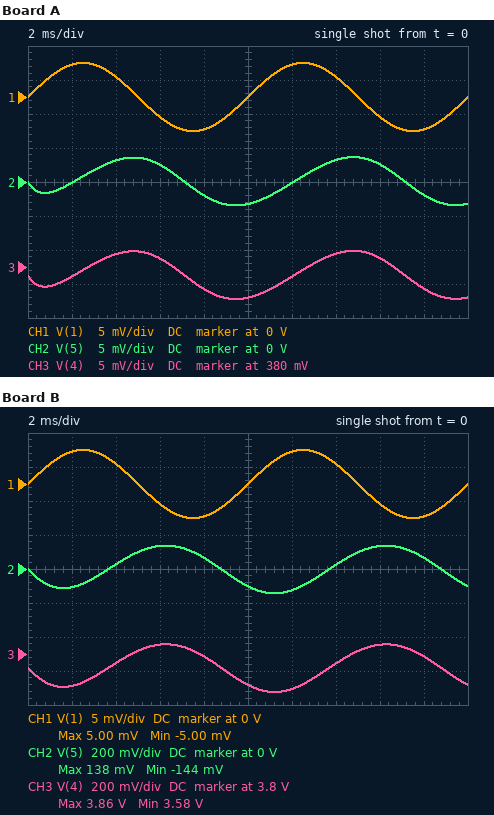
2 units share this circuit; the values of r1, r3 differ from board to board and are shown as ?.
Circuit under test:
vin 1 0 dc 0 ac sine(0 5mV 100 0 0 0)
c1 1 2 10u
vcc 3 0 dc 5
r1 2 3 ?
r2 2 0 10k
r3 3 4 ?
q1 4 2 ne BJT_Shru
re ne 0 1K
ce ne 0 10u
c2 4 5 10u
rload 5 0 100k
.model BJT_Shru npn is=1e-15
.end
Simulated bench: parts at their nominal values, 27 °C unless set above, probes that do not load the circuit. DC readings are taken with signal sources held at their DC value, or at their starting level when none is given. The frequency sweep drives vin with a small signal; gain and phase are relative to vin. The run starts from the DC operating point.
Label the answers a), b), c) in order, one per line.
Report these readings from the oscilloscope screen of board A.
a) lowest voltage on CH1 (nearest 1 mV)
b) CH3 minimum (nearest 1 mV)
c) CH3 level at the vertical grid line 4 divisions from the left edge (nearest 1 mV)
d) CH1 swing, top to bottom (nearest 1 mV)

a) -5 mV
b) 375 mV
c) 377 mV
d) 10 mV
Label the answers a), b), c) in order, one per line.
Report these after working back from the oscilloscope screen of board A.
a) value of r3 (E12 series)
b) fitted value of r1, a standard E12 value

a) 18 kΩ
b) 22 kΩ
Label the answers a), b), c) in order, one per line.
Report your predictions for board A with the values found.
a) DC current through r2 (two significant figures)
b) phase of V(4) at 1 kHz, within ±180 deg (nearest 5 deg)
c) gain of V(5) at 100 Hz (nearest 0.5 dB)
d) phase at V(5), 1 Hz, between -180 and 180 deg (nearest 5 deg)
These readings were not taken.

a) 100 µA
b) -160 deg
c) -3.0 dB
d) 90 deg
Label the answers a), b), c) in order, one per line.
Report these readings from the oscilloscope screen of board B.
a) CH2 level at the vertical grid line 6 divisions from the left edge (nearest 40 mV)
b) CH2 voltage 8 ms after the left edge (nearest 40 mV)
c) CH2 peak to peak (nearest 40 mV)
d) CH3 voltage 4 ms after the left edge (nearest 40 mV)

a) -120 mV
b) 80 mV
c) 280 mV
d) 3.76 V
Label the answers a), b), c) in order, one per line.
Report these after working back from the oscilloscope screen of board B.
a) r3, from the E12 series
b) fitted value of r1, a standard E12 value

a) 6.8 kΩ
b) 47 kΩ
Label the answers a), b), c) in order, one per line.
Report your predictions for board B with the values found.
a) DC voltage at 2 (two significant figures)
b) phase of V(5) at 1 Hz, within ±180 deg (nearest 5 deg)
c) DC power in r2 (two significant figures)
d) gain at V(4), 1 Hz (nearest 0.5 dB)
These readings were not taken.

a) 860 mV
b) -105 deg
c) 74 µW
d) 7.5 dB
